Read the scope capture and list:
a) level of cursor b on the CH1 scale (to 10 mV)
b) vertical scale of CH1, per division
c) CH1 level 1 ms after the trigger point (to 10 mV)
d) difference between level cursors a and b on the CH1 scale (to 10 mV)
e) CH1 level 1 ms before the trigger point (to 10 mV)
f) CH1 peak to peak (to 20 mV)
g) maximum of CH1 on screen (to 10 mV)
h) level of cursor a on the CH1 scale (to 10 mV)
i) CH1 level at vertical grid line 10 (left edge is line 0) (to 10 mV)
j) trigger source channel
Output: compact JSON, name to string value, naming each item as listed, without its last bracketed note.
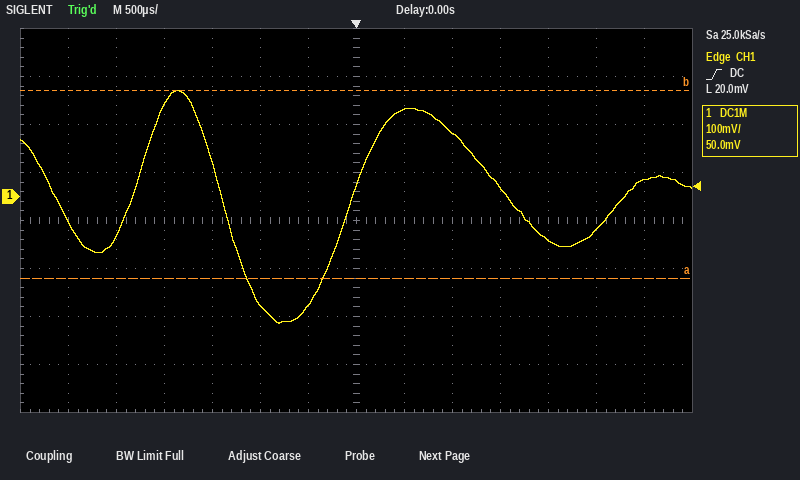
{"level of cursor b on the CH1 scale": "220 mV", "vertical scale of CH1, per division": "100 mV", "CH1 level 1 ms after the trigger point": "130 mV", "difference between level cursors a and b on the CH1 scale": "390 mV", "CH1 level 1 ms before the trigger point": "-230 mV", "CH1 peak to peak": "480 mV", "maximum of CH1 on screen": "220 mV", "level of cursor a on the CH1 scale": "-170 mV", "CH1 level at vertical grid line 10 (left edge is line 0)": "20 mV", "trigger source channel": "CH1"}
